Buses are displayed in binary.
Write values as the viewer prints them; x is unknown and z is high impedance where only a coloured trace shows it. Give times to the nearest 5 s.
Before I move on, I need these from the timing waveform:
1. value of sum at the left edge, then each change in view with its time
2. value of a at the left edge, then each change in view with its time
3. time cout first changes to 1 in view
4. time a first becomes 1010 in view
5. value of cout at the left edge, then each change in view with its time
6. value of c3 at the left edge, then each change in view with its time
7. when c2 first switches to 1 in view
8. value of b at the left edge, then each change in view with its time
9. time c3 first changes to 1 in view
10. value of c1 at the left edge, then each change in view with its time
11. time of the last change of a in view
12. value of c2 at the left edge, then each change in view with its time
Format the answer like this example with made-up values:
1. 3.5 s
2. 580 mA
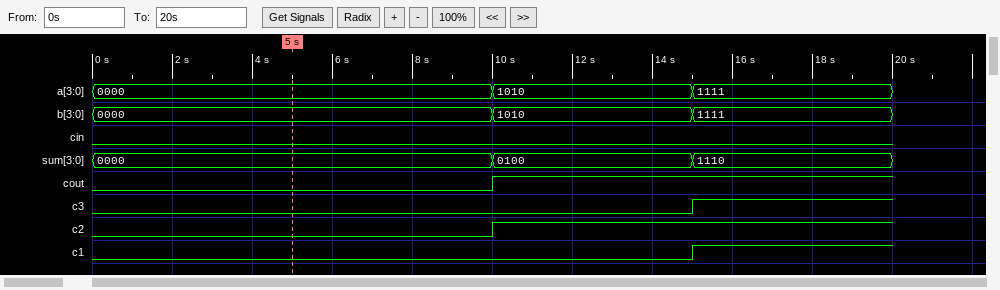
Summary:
1. 0000, 0100 at 10 s, 1110 at 15 s
2. 0000, 1010 at 10 s, 1111 at 15 s
3. 10 s
4. 10 s
5. 0, 1 at 10 s
6. 0, 1 at 15 s
7. 10 s
8. 0000, 1010 at 10 s, 1111 at 15 s
9. 15 s
10. 0, 1 at 15 s
11. 15 s
12. 0, 1 at 10 s
